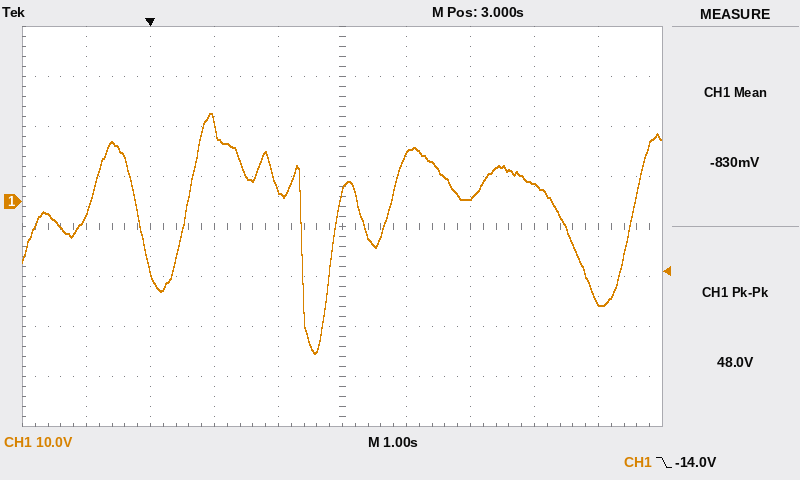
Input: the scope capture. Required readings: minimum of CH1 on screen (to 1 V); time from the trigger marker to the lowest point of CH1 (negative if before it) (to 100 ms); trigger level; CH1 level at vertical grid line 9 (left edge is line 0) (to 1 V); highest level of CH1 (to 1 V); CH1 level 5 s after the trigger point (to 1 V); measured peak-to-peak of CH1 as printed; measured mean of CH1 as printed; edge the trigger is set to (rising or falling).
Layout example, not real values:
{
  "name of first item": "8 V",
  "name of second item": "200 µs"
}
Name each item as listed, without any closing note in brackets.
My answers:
{
  "minimum of CH1 on screen": "-30 V",
  "time from the trigger marker to the lowest point of CH1 (negative if before it)": "+2.6 s",
  "trigger level": "-14.0 V",
  "CH1 level at vertical grid line 9 (left edge is line 0)": "-20 V",
  "highest level of CH1": "18 V",
  "CH1 level 5 s after the trigger point": "1 V",
  "measured peak-to-peak of CH1 as printed": "48.0 V",
  "measured mean of CH1 as printed": "-830 mV",
  "edge the trigger is set to": "falling"
}
